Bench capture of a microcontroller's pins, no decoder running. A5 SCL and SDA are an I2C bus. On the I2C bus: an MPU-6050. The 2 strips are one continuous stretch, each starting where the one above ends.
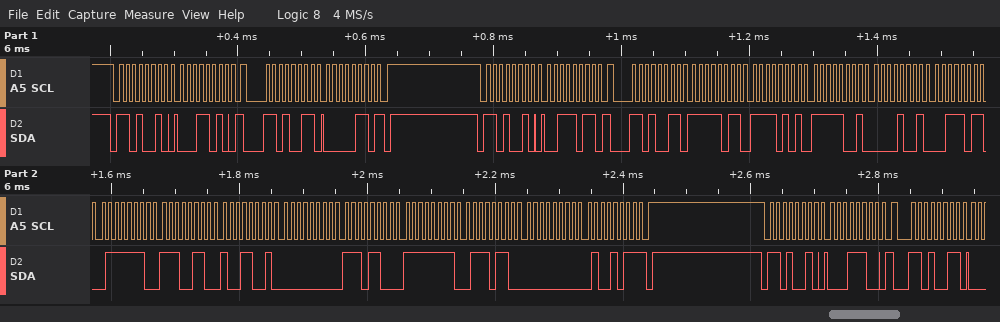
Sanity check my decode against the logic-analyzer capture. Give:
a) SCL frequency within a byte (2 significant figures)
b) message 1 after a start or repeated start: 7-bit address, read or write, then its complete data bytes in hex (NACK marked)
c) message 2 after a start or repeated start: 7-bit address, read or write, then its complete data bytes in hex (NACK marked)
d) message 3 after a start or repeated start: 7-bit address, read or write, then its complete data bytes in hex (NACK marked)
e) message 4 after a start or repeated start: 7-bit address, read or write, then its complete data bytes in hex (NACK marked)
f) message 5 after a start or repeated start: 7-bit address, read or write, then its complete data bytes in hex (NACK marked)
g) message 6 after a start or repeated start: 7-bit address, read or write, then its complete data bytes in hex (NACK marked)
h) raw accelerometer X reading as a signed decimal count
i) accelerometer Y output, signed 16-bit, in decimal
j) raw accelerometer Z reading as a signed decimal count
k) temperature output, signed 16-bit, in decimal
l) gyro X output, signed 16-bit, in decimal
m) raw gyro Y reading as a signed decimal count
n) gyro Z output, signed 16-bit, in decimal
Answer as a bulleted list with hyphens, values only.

- 100 kHz
- 0x69 write: 1A
- 0x69 read: 06 NACK
- 0x69 write: 3B
- 0x69 read: FB F5 F9 09 3B 7E E6 99 00 EC FF 76 00 4B NACK
- 0x69 write: 1C
- 0x69 read
- -1035
- -1783
- 15230
- -6503
- 236
- -138
- 75
